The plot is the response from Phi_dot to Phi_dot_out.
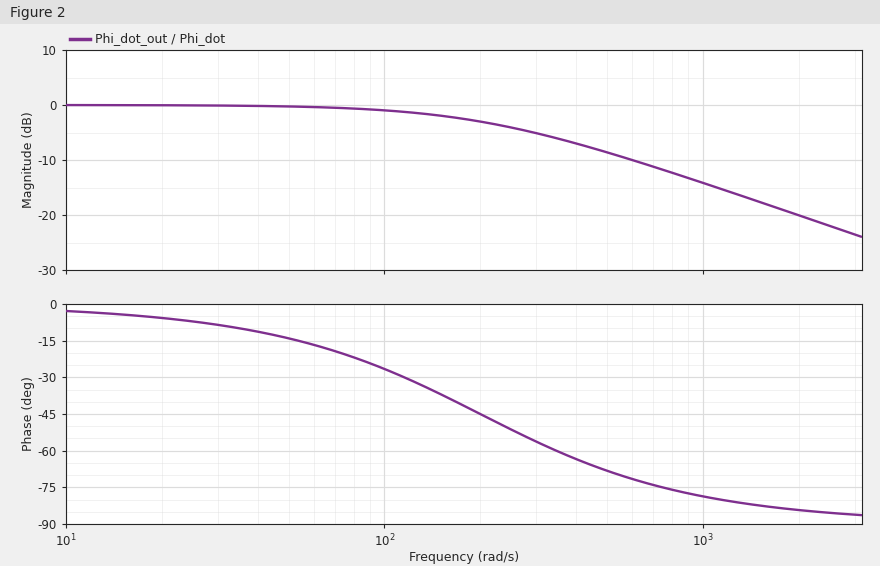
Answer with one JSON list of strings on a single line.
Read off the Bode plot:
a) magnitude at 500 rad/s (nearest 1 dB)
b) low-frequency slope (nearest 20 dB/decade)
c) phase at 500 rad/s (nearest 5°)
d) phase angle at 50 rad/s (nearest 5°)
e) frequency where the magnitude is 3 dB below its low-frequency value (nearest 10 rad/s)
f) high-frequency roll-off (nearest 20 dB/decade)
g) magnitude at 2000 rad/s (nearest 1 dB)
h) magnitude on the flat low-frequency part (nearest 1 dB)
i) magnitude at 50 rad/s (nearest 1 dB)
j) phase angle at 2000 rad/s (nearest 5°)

["-9 dB", "0 dB/decade", "-70°", "-15°", "200 rad/s", "-20 dB/decade", "-20 dB", "0 dB", "0 dB", "-85°"]
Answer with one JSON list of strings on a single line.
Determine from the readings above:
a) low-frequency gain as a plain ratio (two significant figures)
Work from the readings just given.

["1.0"]
